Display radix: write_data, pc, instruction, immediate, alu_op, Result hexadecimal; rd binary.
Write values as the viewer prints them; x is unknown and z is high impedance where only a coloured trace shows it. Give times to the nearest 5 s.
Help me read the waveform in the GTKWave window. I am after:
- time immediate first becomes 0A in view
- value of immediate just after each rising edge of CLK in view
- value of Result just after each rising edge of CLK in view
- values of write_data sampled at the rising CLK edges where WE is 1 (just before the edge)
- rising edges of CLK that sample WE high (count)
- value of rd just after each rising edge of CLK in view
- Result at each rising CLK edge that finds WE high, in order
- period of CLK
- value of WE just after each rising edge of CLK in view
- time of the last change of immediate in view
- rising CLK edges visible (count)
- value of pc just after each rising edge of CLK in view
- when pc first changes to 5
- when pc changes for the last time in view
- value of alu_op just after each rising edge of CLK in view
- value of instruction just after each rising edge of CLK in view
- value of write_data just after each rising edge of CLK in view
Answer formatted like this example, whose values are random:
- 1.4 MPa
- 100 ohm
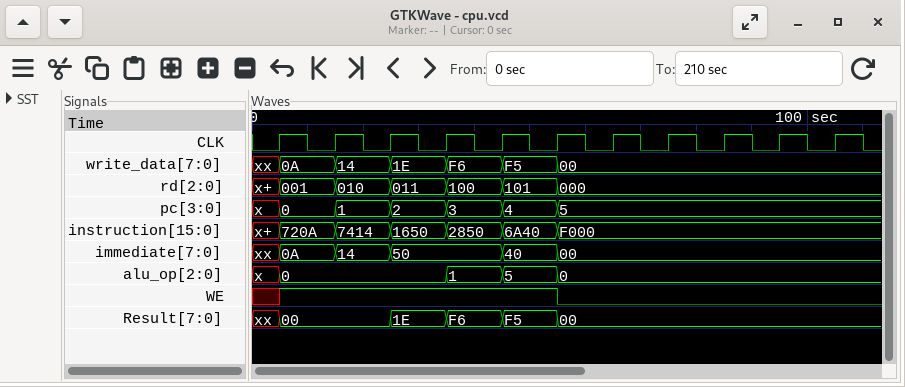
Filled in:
- 5 s
- 0A, 14, 50, 50, 40, 00, 00, 00, 00, 00, 00
- 00, 00, 1E, F6, F5, 00, 00, 00, 00, 00, 00
- 0A, 14, 1E, F6, F5
- 5
- 001, 010, 011, 100, 101, 000, 000, 000, 000, 000, 000
- 00, 00, 1E, F6, F5
- 10 s
- 1 1 1 1 1 0 0 0 0 0 0
- 55 s
- 11
- 0, 1, 2, 3, 4, 5, 5, 5, 5, 5, 5
- 55 s
- 55 s
- 0, 0, 0, 1, 5, 0, 0, 0, 0, 0, 0
- 720A, 7414, 1650, 2850, 6A40, F000, F000, F000, F000, F000, F000
- 0A, 14, 1E, F6, F5, 00, 00, 00, 00, 00, 00
